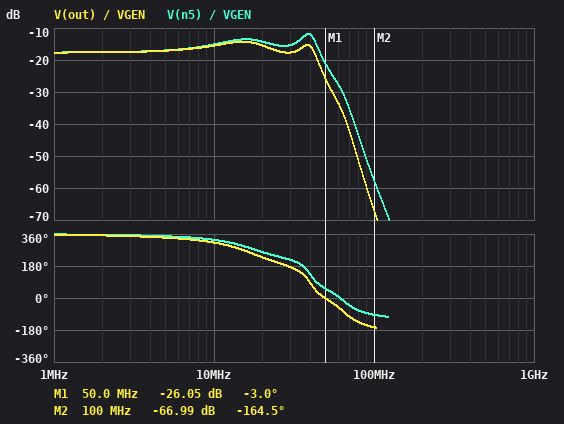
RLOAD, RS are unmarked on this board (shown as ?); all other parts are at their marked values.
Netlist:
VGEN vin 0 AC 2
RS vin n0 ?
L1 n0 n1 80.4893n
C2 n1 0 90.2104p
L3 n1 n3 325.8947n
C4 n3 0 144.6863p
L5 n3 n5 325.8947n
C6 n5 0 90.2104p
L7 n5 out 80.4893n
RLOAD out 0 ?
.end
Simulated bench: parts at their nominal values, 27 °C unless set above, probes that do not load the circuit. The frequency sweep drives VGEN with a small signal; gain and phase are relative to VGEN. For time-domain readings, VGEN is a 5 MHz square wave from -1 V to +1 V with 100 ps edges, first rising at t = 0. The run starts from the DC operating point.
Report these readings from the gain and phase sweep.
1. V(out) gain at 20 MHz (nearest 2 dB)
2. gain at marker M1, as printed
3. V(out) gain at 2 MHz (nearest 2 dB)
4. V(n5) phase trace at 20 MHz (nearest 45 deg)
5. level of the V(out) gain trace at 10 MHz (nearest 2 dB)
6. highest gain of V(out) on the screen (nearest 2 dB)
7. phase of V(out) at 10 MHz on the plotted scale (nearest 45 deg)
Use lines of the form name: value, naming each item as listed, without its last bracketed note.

V(out) gain at 20 MHz: -16 dB
gain at marker M1, as printed: -26.05 dB
V(out) gain at 2 MHz: -18 dB
V(n5) phase trace at 20 MHz: 270 deg
level of the V(out) gain trace at 10 MHz: -16 dB
highest gain of V(out) on the screen: -14 dB
phase of V(out) at 10 MHz on the plotted scale: 315 deg
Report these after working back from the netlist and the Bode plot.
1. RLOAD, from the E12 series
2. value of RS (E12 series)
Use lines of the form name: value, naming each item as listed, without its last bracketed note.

RLOAD, from the E12 series: 18 Ω
value of RS: 120 Ω
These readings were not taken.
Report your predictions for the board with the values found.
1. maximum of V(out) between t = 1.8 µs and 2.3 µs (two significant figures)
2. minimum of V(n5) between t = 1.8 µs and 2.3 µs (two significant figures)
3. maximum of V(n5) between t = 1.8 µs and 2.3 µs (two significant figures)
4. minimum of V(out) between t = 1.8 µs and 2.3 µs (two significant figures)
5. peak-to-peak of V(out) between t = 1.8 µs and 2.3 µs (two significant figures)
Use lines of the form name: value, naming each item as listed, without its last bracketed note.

maximum of V(out) between t = 1.8 µs and 2.3 µs: 230 mV
minimum of V(n5) between t = 1.8 µs and 2.3 µs: -270 mV
maximum of V(n5) between t = 1.8 µs and 2.3 µs: 270 mV
minimum of V(out) between t = 1.8 µs and 2.3 µs: -230 mV
peak-to-peak of V(out) between t = 1.8 µs and 2.3 µs: 450 mV
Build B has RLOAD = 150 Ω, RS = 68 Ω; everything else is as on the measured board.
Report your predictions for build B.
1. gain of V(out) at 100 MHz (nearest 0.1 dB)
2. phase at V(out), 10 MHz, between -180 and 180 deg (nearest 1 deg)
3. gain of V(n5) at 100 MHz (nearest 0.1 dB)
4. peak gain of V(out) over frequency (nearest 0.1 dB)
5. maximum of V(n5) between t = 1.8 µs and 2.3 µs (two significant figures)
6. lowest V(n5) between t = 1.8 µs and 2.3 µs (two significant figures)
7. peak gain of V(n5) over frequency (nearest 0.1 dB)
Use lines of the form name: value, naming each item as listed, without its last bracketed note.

gain of V(out) at 100 MHz: -56.8 dB
phase at V(out), 10 MHz, between -180 and 180 deg: -63 deg
gain of V(n5) at 100 MHz: -56.3 dB
peak gain of V(out) over frequency: -2.7 dB
maximum of V(n5) between t = 1.8 µs and 2.3 µs: 820 mV
lowest V(n5) between t = 1.8 µs and 2.3 µs: -820 mV
peak gain of V(n5) over frequency: -2.6 dB
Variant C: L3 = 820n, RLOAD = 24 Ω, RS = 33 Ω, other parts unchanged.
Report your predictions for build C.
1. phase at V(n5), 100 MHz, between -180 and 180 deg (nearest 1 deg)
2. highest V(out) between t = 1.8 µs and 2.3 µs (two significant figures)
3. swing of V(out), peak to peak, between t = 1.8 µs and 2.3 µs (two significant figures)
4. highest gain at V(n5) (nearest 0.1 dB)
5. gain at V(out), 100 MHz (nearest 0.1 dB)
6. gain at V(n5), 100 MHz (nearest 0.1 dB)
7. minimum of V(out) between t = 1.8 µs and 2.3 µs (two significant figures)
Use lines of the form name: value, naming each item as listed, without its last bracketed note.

phase at V(n5), 100 MHz, between -180 and 180 deg: -122 deg
highest V(out) between t = 1.8 µs and 2.3 µs: 420 mV
swing of V(out), peak to peak, between t = 1.8 µs and 2.3 µs: 840 mV
highest gain at V(n5): -7.5 dB
gain at V(out), 100 MHz: -65.5 dB
gain at V(n5), 100 MHz: -58.2 dB
minimum of V(out) between t = 1.8 µs and 2.3 µs: -420 mV
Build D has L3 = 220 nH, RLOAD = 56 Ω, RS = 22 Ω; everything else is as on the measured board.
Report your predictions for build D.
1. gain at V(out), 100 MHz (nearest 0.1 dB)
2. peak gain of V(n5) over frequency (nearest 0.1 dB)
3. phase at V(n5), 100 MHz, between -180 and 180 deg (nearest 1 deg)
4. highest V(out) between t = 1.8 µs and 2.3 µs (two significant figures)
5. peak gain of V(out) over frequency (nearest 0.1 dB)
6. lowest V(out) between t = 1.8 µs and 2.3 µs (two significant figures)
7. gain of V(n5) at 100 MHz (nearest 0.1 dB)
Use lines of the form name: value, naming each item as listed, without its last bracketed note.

gain at V(out), 100 MHz: -47.6 dB
peak gain of V(n5) over frequency: -1.8 dB
phase at V(n5), 100 MHz, between -180 and 180 deg: -131 deg
highest V(out) between t = 1.8 µs and 2.3 µs: 1.0 V
peak gain of V(out) over frequency: -2.1 dB
lowest V(out) between t = 1.8 µs and 2.3 µs: -1.0 V
gain of V(n5) at 100 MHz: -45.0 dB
